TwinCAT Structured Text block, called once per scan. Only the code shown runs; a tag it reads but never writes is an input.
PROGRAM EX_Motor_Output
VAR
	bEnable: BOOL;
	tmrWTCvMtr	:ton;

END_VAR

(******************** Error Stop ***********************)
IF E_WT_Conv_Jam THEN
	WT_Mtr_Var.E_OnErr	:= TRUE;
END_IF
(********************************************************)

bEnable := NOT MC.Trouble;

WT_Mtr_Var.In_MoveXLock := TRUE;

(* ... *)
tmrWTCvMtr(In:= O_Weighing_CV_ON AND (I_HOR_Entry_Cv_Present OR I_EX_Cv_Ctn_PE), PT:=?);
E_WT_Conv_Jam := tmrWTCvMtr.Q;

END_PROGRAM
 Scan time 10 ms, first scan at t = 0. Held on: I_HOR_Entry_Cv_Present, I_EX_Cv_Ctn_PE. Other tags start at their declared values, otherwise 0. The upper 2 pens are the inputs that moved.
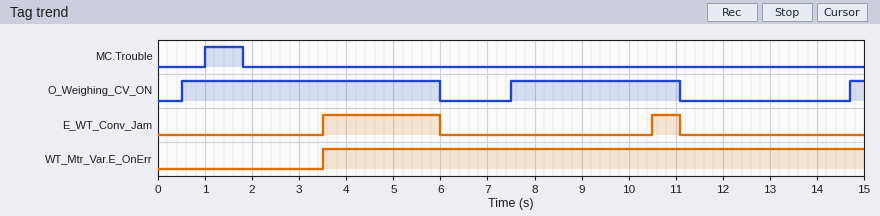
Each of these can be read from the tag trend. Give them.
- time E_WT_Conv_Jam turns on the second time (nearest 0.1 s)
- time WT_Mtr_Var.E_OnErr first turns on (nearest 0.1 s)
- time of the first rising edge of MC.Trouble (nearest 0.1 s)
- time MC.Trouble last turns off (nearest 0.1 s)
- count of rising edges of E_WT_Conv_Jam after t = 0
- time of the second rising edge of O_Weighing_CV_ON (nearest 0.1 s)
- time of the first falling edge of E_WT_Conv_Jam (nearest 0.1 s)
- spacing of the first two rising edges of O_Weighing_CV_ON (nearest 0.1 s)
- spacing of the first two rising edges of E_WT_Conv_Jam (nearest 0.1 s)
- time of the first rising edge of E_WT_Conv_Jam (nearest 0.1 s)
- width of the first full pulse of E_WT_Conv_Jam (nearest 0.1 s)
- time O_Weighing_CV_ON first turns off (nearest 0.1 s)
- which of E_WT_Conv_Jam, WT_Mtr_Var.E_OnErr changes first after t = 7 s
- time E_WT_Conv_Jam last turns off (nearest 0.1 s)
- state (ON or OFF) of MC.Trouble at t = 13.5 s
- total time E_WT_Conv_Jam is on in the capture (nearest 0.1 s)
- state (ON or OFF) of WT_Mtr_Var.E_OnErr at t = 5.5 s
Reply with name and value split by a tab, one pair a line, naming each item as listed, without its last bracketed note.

time E_WT_Conv_Jam turns on the second time	10.5 s
time WT_Mtr_Var.E_OnErr first turns on	3.5 s
time of the first rising edge of MC.Trouble	1.0 s
time MC.Trouble last turns off	1.8 s
count of rising edges of E_WT_Conv_Jam after t = 0	2
time of the second rising edge of O_Weighing_CV_ON	7.5 s
time of the first falling edge of E_WT_Conv_Jam	6.0 s
spacing of the first two rising edges of O_Weighing_CV_ON	7.0 s
spacing of the first two rising edges of E_WT_Conv_Jam	7.0 s
time of the first rising edge of E_WT_Conv_Jam	3.5 s
width of the first full pulse of E_WT_Conv_Jam	2.5 s
time O_Weighing_CV_ON first turns off	6.0 s
which of E_WT_Conv_Jam, WT_Mtr_Var.E_OnErr changes first after t = 7 s	E_WT_Conv_Jam
time E_WT_Conv_Jam last turns off	11.1 s
state (ON or OFF) of MC.Trouble at t = 13.5 s	OFF
total time E_WT_Conv_Jam is on in the capture	3.1 s
state (ON or OFF) of WT_Mtr_Var.E_OnErr at t = 5.5 s	ON
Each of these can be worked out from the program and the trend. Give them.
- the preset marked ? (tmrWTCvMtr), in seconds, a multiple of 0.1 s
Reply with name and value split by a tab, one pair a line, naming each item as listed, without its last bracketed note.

the preset marked ? (tmrWTCvMtr), in seconds, a multiple of 0.1 s	3.0 s
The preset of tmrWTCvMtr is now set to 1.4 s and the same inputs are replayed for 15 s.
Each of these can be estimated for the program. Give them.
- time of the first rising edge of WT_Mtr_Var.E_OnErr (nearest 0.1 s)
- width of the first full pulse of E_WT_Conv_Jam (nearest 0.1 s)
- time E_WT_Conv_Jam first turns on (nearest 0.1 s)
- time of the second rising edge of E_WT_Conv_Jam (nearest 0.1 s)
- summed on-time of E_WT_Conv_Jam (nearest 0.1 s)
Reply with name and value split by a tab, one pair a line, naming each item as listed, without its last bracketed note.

time of the first rising edge of WT_Mtr_Var.E_OnErr	1.9 s
width of the first full pulse of E_WT_Conv_Jam	4.1 s
time E_WT_Conv_Jam first turns on	1.9 s
time of the second rising edge of E_WT_Conv_Jam	8.9 s
summed on-time of E_WT_Conv_Jam	6.3 s
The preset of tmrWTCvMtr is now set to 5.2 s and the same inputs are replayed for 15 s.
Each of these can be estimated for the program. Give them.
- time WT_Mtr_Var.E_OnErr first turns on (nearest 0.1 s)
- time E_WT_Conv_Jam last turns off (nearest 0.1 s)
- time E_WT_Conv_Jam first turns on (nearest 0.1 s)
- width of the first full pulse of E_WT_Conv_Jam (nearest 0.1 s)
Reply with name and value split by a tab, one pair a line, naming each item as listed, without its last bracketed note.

time WT_Mtr_Var.E_OnErr first turns on	5.7 s
time E_WT_Conv_Jam last turns off	6.0 s
time E_WT_Conv_Jam first turns on	5.7 s
width of the first full pulse of E_WT_Conv_Jam	0.3 s
